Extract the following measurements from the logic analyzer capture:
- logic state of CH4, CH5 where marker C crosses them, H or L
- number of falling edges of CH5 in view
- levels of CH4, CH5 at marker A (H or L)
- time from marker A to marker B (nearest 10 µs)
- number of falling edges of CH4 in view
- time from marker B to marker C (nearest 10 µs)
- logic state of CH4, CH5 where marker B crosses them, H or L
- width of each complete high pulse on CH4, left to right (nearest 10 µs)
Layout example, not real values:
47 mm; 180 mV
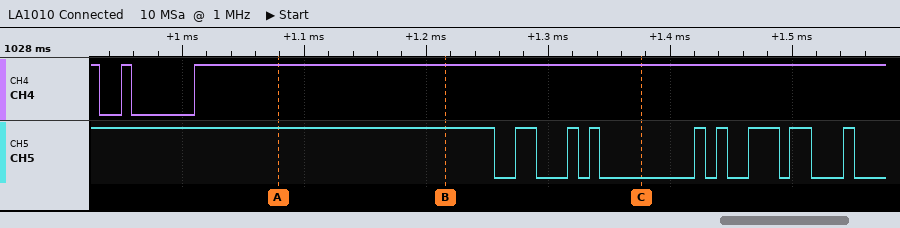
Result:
CH4=H, CH5=L; 9; CH4=H, CH5=H; 140 µs; 2; 160 µs; CH4=H, CH5=H; 10 µs
